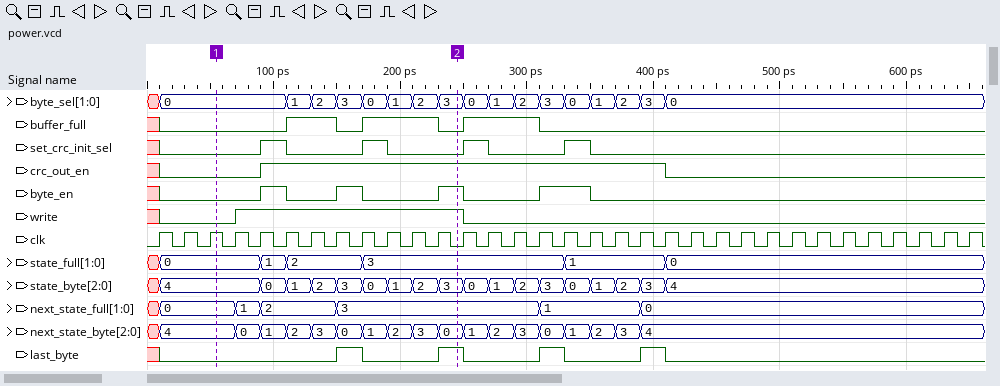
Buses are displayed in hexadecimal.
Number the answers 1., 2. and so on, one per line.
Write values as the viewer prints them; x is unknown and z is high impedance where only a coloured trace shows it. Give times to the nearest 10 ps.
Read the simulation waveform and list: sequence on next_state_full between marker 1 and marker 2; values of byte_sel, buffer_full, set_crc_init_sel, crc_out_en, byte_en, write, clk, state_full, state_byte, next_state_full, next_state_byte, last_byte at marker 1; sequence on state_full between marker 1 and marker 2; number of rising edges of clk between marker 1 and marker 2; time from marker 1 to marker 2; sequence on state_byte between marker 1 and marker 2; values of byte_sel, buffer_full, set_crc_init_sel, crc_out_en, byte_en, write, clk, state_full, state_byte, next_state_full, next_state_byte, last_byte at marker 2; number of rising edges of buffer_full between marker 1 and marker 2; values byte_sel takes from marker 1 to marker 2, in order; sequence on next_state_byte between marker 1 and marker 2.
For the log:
1. 0, 1, 2, 3
2. byte_sel=0, buffer_full=0, set_crc_init_sel=0, crc_out_en=0, byte_en=0, write=0, clk=1, state_full=0, state_byte=4, next_state_full=0, next_state_byte=4, last_byte=0
3. 0, 1, 2, 3
4. 9
5. 190 ps
6. 4, 0, 1, 2, 3, 0, 1, 2, 3
7. byte_sel=3, buffer_full=0, set_crc_init_sel=0, crc_out_en=1, byte_en=1, write=1, clk=0, state_full=3, state_byte=3, next_state_full=3, next_state_byte=0, last_byte=1
8. 2
9. 0, 1, 2, 3, 0, 1, 2, 3
10. 4, 0, 1, 2, 3, 0, 1, 2, 3, 0
